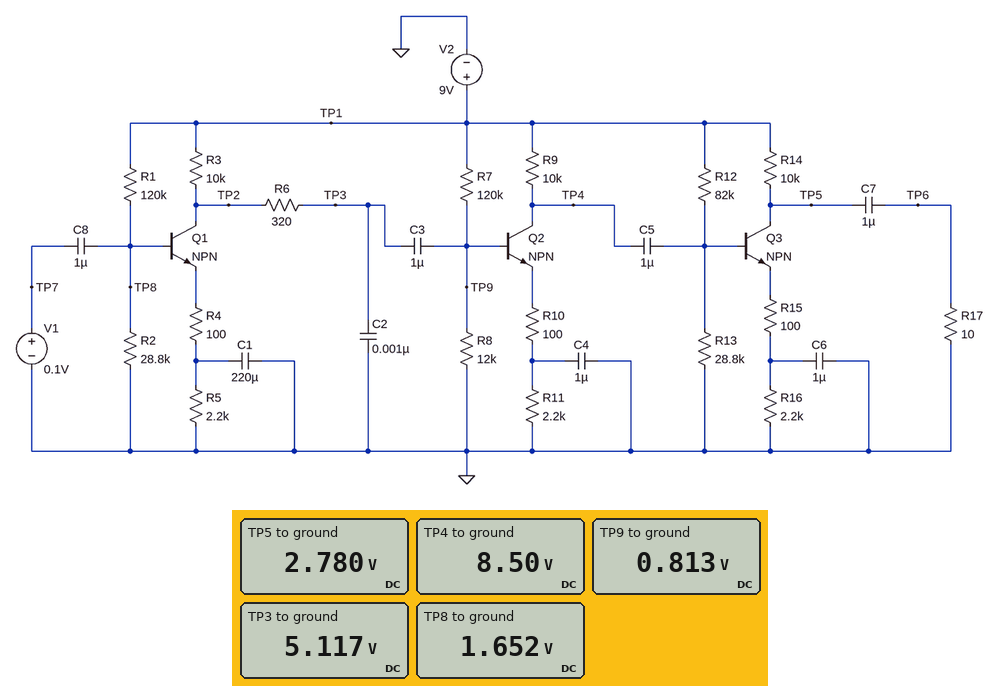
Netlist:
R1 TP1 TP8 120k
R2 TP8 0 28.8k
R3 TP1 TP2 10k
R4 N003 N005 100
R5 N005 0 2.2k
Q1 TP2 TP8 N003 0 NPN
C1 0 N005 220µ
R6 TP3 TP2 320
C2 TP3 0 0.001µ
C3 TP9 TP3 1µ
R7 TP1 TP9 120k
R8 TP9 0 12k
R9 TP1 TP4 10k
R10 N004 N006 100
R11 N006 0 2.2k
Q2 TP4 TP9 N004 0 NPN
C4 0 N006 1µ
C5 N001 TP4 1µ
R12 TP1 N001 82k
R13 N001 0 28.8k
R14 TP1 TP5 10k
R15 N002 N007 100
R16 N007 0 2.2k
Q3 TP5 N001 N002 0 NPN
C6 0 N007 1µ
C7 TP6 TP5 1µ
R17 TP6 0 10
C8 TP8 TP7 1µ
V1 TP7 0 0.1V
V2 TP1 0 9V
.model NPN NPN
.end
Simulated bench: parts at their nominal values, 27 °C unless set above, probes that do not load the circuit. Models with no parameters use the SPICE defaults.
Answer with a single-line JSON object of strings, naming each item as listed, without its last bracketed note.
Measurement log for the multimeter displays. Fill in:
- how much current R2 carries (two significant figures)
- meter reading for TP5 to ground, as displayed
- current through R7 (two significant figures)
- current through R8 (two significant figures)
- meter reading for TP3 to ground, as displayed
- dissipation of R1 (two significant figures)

{"how much current R2 carries": "57 µA", "meter reading for TP5 to ground, as displayed": "2.780 V", "current through R7": "68 µA", "current through R8": "68 µA", "meter reading for TP3 to ground, as displayed": "5.117 V", "dissipation of R1": "450 µW"}
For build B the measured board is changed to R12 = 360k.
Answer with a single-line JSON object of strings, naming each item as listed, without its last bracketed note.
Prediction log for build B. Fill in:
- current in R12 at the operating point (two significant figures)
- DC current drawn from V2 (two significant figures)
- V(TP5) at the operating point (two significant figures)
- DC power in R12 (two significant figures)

{"current in R12 at the operating point": "23 µA", "DC current drawn from V2": "600 µA", "V(TP5) at the operating point": "8.9 V", "DC power in R12": "190 µW"}
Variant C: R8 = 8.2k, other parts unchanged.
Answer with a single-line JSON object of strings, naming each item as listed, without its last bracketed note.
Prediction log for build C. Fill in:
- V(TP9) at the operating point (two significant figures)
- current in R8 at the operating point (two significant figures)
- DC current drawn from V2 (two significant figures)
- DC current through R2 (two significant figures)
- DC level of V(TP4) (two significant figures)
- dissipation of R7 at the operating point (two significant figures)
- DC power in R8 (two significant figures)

{"V(TP9) at the operating point": "580 mV", "current in R8 at the operating point": "70 µA", "DC current drawn from V2": "1.2 mA", "DC current through R2": "57 µA", "DC level of V(TP4)": "9.0 V", "dissipation of R7 at the operating point": "590 µW", "DC power in R8": "40 µW"}
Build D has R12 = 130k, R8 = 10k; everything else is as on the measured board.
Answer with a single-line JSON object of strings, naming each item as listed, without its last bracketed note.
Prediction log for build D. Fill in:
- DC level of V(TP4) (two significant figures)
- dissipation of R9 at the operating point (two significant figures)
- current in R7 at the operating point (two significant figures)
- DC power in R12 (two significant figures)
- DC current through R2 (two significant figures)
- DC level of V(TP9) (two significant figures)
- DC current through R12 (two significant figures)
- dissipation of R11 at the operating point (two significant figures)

{"DC level of V(TP4)": "8.9 V", "dissipation of R9 at the operating point": "1.6 µW", "current in R7 at the operating point": "69 µA", "DC power in R12": "430 µW", "DC current through R2": "57 µA", "DC level of V(TP9)": "690 mV", "DC current through R12": "57 µA", "dissipation of R11 at the operating point": "370 nW"}
